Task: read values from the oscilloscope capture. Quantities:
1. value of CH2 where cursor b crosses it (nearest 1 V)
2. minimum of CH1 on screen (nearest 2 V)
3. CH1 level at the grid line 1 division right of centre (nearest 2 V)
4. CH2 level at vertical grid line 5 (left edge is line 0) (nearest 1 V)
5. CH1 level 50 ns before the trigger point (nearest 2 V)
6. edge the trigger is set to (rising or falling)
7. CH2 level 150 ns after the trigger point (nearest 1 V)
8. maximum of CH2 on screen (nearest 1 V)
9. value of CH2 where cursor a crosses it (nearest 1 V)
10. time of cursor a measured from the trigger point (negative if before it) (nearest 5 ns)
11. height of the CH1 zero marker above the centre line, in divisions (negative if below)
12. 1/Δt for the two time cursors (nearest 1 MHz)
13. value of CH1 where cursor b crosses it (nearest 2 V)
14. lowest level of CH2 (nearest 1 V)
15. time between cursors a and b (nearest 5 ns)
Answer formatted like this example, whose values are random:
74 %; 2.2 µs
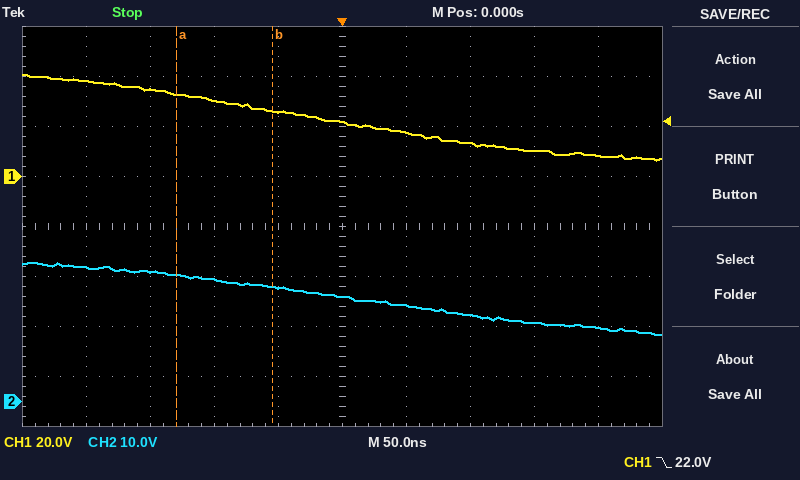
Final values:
23 V; 6 V; 18 V; 21 V; 26 V; falling; 16 V; 28 V; 25 V; -130 ns; +1.0 div; 13 MHz; 26 V; 13 V; 75 ns
